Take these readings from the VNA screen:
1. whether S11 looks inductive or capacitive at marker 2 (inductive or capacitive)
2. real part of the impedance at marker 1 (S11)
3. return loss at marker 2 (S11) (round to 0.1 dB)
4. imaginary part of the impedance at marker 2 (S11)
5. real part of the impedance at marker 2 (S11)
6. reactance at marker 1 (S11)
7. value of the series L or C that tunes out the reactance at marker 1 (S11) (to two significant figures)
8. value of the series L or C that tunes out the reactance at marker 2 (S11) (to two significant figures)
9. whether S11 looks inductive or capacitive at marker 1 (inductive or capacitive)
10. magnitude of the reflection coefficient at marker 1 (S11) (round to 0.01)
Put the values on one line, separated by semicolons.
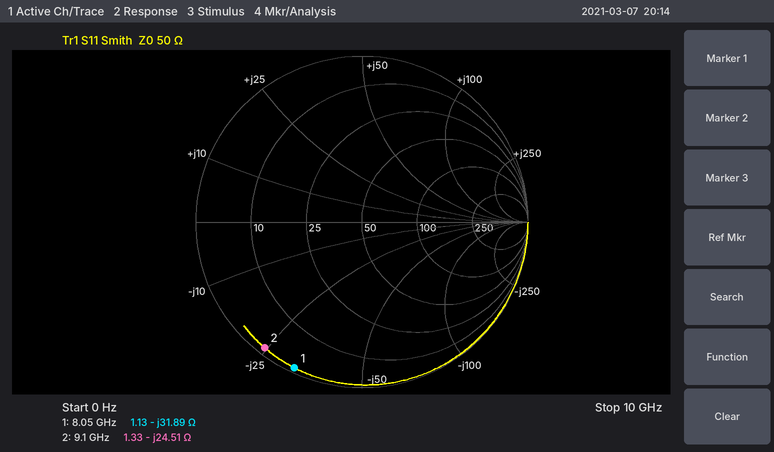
capacitive; 1.13 Ω; 0.4 dB; -24.51 Ω; 1.33 Ω; -31.89 Ω; 630 pH; 430 pH; capacitive; 0.97
